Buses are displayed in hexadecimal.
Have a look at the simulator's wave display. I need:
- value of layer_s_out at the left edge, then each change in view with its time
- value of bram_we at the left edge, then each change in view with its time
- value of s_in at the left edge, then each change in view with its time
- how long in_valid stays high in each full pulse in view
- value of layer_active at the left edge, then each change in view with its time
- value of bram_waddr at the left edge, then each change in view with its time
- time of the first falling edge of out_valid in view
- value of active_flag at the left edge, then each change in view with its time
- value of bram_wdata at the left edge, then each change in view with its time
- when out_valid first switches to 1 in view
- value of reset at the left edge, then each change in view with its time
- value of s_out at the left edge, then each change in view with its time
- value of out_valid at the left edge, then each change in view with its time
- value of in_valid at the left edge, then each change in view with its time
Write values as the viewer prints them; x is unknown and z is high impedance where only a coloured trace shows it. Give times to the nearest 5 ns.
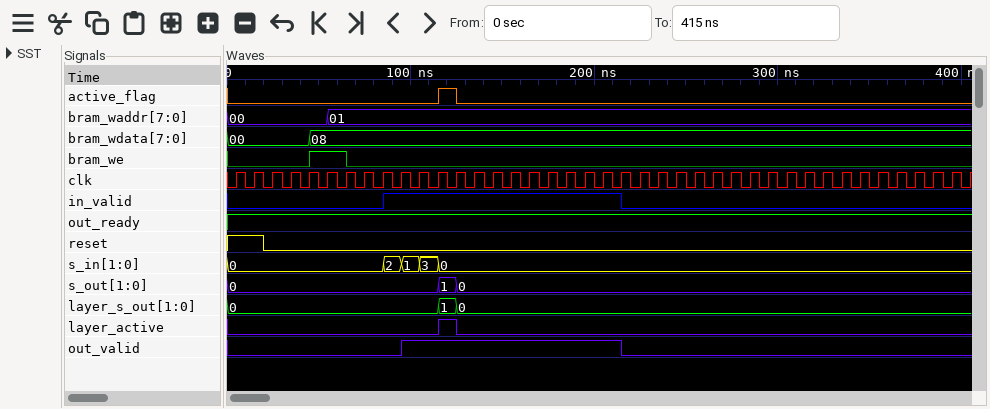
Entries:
0, 1 at 115 ns, 0 at 125 ns
0, 1 at 45 ns, 0 at 65 ns
0, 2 at 85 ns, 1 at 95 ns, 3 at 105 ns, 0 at 115 ns
130 ns
0, 1 at 115 ns, 0 at 125 ns
00, 01 at 55 ns
215 ns
0, 1 at 115 ns, 0 at 125 ns
00, 08 at 45 ns
95 ns
1, 0 at 20 ns
0, 1 at 115 ns, 0 at 125 ns
0, 1 at 95 ns, 0 at 215 ns
0, 1 at 85 ns, 0 at 215 ns
